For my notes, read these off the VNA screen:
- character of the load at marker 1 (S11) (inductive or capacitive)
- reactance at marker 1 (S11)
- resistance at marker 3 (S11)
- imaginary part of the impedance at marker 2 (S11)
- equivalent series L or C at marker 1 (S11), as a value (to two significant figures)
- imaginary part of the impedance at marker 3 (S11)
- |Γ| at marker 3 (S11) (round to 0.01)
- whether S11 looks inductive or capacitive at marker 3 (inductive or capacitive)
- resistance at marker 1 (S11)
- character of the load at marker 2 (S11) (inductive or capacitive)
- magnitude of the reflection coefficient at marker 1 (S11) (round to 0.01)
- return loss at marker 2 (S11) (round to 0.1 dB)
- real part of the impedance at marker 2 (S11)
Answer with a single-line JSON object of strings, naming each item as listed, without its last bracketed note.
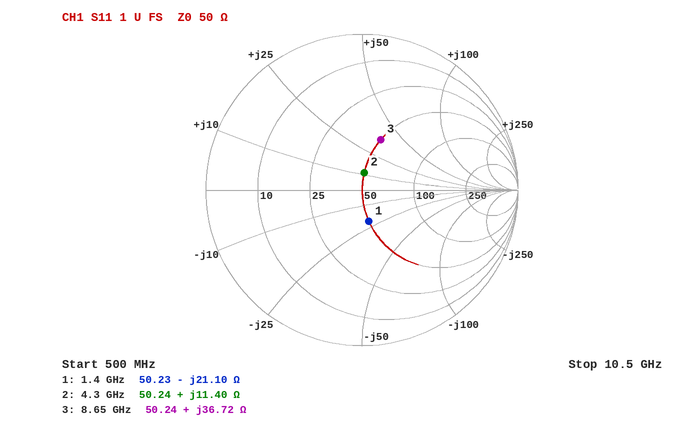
{"character of the load at marker 1 (S11)": "capacitive", "reactance at marker 1": "-21.10 Ω", "resistance at marker 3": "50.24 Ω", "imaginary part of the impedance at marker 2": "+11.40 Ω", "equivalent series L or C at marker 1 (S11), as a value": "5.4 pF", "imaginary part of the impedance at marker 3": "+36.72 Ω", "|Γ| at marker 3 (S11)": "0.34", "whether S11 looks inductive or capacitive at marker 3": "inductive", "resistance at marker 1": "50.23 Ω", "character of the load at marker 2 (S11)": "inductive", "magnitude of the reflection coefficient at marker 1 (S11)": "0.21", "return loss at marker 2 (S11)": "18.9 dB", "real part of the impedance at marker 2": "50.24 Ω"}
